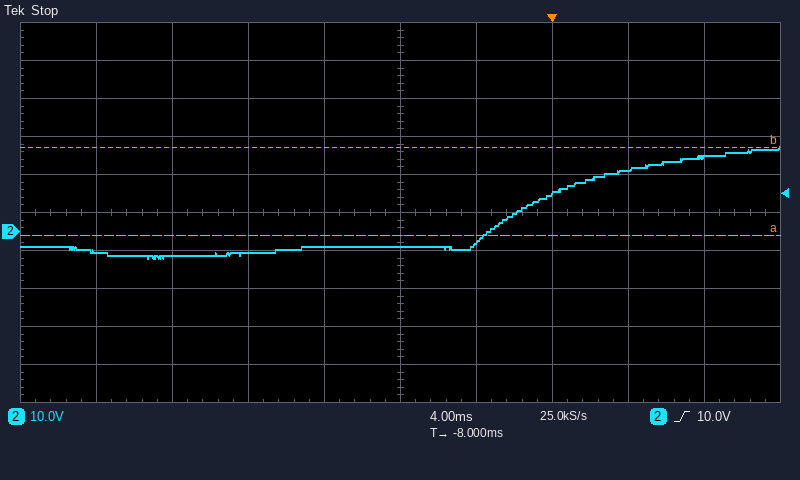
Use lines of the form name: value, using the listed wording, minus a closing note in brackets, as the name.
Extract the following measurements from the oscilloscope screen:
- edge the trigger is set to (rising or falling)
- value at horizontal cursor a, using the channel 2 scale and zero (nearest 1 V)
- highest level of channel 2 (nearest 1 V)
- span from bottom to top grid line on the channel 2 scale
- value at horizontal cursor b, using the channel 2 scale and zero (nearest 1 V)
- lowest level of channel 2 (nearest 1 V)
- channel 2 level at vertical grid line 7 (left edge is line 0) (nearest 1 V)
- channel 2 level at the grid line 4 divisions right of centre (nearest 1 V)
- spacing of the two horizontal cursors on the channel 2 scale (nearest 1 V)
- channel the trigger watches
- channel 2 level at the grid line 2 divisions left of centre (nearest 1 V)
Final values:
edge the trigger is set to: rising
value at horizontal cursor a, using the channel 2 scale and zero: -1 V
highest level of channel 2: 22 V
span from bottom to top grid line on the channel 2 scale: 100 V
value at horizontal cursor b, using the channel 2 scale and zero: 22 V
lowest level of channel 2: -7 V
channel 2 level at vertical grid line 7 (left edge is line 0): 10 V
channel 2 level at the grid line 4 divisions right of centre: 20 V
spacing of the two horizontal cursors on the channel 2 scale: 23 V
channel the trigger watches: channel 2
channel 2 level at the grid line 2 divisions left of centre: -6 V
